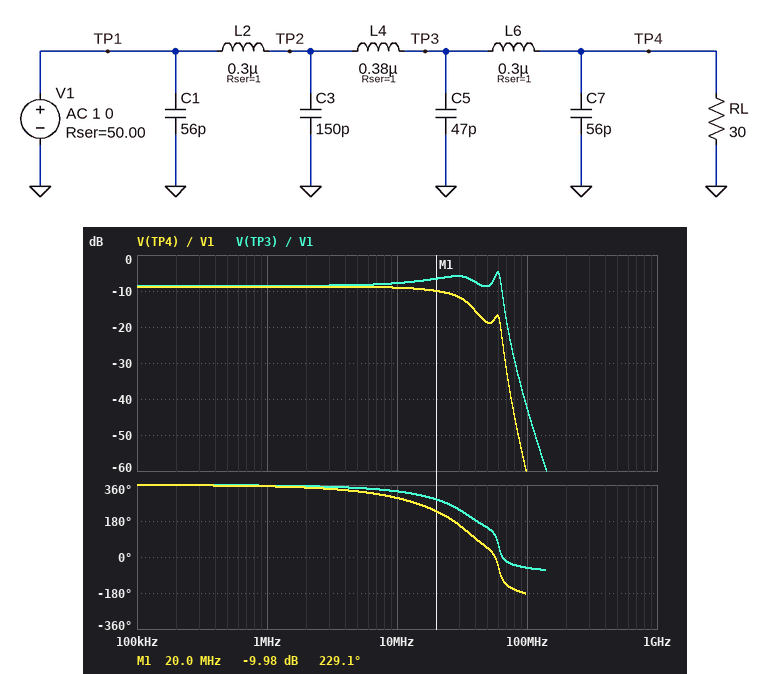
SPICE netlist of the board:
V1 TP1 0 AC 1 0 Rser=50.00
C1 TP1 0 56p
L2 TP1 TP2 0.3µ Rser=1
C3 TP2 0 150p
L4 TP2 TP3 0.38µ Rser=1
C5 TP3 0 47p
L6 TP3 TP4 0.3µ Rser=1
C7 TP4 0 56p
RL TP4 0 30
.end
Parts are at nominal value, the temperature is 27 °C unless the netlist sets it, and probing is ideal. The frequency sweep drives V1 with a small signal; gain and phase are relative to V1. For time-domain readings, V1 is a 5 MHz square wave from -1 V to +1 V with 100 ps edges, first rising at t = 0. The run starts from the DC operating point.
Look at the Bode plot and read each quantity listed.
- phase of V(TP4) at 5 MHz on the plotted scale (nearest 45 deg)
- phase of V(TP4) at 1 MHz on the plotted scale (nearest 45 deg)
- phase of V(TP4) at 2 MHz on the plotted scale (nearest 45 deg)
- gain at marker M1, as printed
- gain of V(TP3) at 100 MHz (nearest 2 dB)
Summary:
315 deg
360 deg
360 deg
-9.98 dB
-42 dB
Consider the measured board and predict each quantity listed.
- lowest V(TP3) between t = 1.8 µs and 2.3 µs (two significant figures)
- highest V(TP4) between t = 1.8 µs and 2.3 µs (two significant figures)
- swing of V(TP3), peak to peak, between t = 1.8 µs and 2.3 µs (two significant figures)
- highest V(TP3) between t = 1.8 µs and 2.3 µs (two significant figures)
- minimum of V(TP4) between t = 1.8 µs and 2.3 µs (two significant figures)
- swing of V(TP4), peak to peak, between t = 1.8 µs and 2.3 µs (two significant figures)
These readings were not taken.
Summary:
-630 mV
380 mV
1.3 V
630 mV
-380 mV
760 mV
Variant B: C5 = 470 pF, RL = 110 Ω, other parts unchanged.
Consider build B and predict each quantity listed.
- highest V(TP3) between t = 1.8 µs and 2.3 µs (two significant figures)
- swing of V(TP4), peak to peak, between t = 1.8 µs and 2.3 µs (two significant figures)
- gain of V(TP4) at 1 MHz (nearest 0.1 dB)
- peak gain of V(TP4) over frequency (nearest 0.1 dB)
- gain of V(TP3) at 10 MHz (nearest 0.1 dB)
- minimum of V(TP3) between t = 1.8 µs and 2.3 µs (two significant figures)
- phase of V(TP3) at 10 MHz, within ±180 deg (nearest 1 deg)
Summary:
670 mV
1.3 V
-3.5 dB
-3.4 dB
-6.3 dB
-670 mV
-92 deg
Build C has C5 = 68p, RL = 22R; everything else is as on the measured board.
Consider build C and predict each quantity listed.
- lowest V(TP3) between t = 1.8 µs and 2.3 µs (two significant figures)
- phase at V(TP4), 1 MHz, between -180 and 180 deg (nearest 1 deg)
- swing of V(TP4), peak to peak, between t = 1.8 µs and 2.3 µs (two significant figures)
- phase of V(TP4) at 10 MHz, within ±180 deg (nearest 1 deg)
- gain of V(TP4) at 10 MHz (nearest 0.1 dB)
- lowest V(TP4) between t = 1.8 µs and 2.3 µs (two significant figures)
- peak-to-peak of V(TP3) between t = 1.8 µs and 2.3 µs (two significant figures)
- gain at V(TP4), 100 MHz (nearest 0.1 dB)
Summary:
-720 mV
-7 deg
640 mV
-67 deg
-10.9 dB
-320 mV
1.4 V
-67.2 dB
